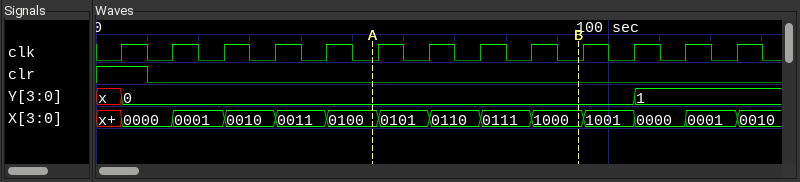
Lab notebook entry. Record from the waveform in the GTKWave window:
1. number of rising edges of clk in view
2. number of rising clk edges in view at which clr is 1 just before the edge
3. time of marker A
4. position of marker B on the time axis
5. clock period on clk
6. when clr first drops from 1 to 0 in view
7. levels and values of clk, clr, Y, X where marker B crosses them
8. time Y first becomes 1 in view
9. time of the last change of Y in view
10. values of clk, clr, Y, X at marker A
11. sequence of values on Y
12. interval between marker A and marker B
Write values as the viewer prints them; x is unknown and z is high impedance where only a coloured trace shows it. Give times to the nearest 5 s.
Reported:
13
1
55 s
95 s
10 s
10 s
clk=0, clr=0, Y=0, X=1000
105 s
105 s
clk=0, clr=0, Y=0, X=0100
x, 0, 1
40 s
